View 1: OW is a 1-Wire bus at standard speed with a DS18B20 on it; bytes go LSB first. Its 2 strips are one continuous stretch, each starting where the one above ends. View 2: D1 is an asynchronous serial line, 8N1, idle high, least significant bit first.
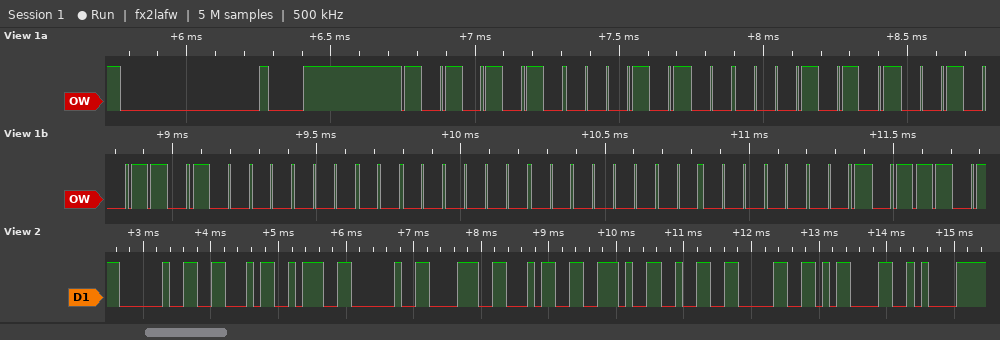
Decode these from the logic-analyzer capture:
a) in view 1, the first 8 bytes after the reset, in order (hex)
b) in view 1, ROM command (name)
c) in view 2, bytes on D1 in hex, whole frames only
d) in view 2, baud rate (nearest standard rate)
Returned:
55 28 A8 64 01 00 00 80
Match ROM
20 46 3A 20 38 34 2E 32 30 0D 0A
9600 baud
